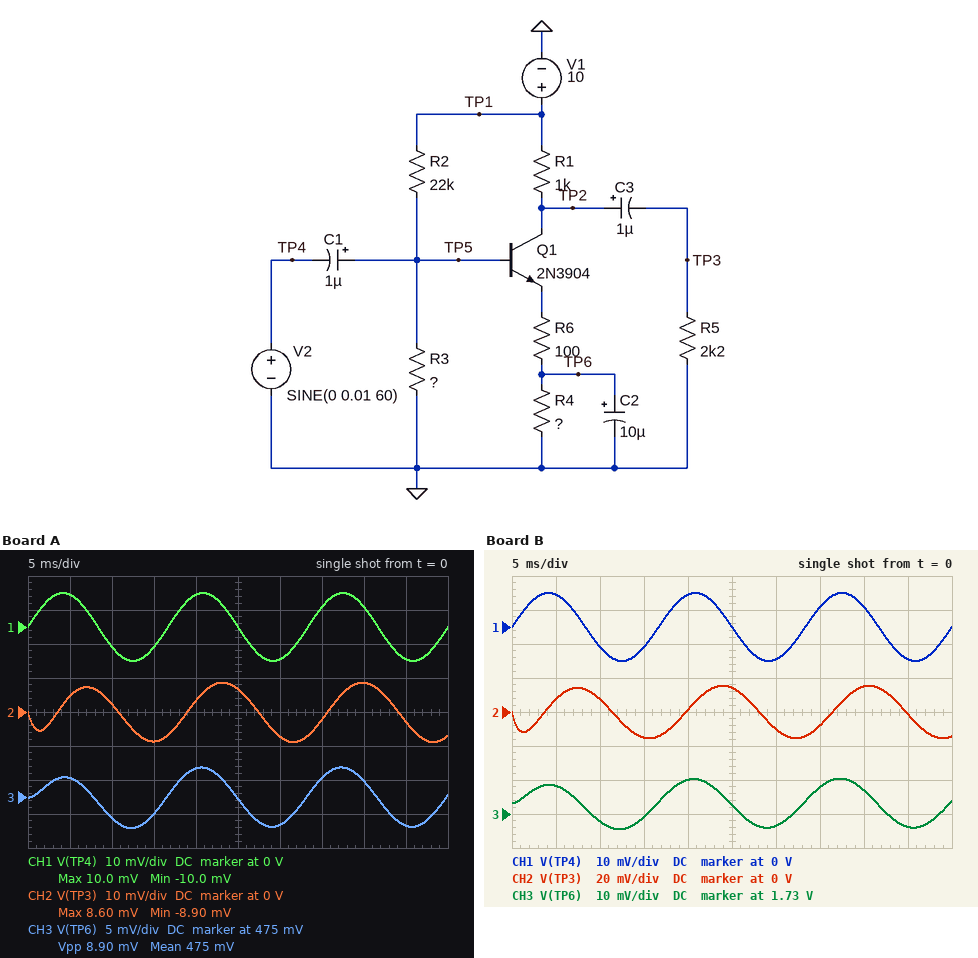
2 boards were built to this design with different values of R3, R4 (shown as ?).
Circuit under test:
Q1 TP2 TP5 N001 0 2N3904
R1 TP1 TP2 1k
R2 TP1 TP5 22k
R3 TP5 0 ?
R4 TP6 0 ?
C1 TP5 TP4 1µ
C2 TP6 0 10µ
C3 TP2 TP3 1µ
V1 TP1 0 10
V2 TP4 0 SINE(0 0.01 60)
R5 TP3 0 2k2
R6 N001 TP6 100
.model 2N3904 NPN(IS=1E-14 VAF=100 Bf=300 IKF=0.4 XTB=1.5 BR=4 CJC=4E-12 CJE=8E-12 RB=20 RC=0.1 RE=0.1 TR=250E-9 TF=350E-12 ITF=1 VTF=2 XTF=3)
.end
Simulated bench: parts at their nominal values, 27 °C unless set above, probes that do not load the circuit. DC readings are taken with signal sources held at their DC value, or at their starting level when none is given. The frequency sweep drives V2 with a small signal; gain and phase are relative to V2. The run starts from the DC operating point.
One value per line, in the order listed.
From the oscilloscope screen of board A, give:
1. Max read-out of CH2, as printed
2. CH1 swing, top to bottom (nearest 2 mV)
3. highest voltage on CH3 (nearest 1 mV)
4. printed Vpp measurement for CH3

8.60 mV
20 mV
479 mV
8.90 mV
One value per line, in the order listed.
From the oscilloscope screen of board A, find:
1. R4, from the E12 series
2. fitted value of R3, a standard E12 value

3.3 kΩ
2.7 kΩ
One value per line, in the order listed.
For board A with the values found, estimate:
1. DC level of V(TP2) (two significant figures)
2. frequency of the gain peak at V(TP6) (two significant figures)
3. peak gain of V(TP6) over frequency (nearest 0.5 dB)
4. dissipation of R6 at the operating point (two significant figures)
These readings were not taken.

9.9 V
64 Hz
-7.0 dB
2.1 µW
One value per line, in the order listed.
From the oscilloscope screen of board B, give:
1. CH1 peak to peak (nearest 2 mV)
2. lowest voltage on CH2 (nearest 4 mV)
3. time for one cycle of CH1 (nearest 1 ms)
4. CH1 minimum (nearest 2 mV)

20 mV
-16 mV
17 ms
-10 mV
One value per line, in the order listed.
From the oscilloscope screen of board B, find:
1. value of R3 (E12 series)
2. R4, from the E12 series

8.2 kΩ
680 Ω
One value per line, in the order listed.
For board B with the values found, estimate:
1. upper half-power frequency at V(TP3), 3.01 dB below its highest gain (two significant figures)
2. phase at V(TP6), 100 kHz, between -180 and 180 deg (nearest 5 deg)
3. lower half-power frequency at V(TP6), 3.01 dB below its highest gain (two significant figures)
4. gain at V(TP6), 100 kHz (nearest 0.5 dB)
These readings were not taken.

89 MHz
-90 deg
21 Hz
-57.0 dB
